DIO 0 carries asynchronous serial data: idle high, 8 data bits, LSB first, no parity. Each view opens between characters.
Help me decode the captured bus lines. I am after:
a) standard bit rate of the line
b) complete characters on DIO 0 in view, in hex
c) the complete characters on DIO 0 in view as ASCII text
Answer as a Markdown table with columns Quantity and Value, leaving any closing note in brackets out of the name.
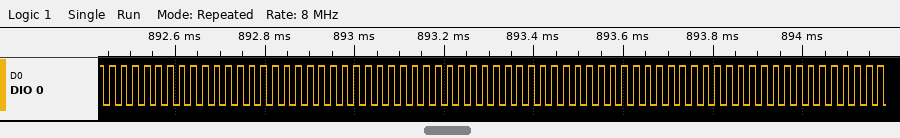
| Quantity | Value |
|---|---|
| standard bit rate of the line | 74880 baud |
| complete characters on DIO 0 in view, in hex | 55, 55, 55, 55, 55, 55, 55, 55, 55, 55, 55, 55, 55 |
| the complete characters on DIO 0 in view as ASCII text | "UUUUUUUUUUUUU" |
